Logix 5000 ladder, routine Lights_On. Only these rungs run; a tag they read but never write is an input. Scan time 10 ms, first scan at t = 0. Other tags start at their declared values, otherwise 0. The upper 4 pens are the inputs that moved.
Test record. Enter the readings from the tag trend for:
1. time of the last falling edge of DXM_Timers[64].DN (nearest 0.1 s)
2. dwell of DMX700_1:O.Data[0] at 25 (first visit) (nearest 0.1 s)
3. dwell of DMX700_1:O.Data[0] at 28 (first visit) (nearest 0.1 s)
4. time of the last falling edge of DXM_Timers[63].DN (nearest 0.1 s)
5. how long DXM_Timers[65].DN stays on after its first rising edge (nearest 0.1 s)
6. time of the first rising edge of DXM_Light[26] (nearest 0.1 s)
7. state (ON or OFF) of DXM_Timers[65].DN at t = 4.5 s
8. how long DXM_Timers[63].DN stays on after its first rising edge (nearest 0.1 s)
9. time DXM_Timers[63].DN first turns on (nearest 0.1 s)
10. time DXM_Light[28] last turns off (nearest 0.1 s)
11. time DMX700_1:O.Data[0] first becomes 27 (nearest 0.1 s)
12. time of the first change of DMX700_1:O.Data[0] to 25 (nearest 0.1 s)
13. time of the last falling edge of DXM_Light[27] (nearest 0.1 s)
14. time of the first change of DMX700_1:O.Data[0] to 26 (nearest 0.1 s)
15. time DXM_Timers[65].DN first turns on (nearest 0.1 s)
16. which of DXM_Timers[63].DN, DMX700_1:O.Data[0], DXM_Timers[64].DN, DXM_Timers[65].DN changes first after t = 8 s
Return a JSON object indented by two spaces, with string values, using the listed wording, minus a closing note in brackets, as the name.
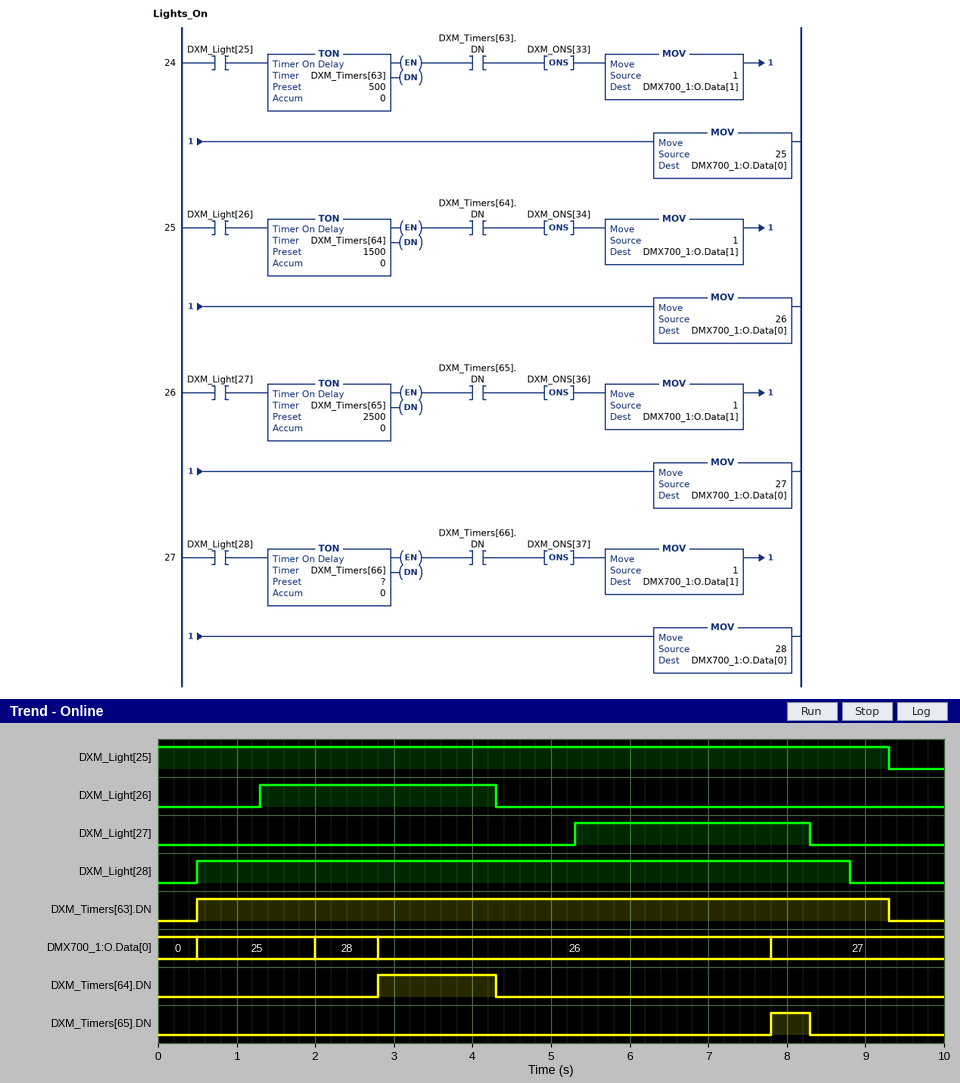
{
  "time of the last falling edge of DXM_Timers[64].DN": "4.3 s",
  "dwell of DMX700_1:O.Data[0] at 25 (first visit)": "1.5 s",
  "dwell of DMX700_1:O.Data[0] at 28 (first visit)": "0.8 s",
  "time of the last falling edge of DXM_Timers[63].DN": "9.3 s",
  "how long DXM_Timers[65].DN stays on after its first rising edge": "0.5 s",
  "time of the first rising edge of DXM_Light[26]": "1.3 s",
  "state (ON or OFF) of DXM_Timers[65].DN at t = 4.5 s": "OFF",
  "how long DXM_Timers[63].DN stays on after its first rising edge": "8.8 s",
  "time DXM_Timers[63].DN first turns on": "0.5 s",
  "time DXM_Light[28] last turns off": "8.8 s",
  "time DMX700_1:O.Data[0] first becomes 27": "7.8 s",
  "time of the first change of DMX700_1:O.Data[0] to 25": "0.5 s",
  "time of the last falling edge of DXM_Light[27]": "8.3 s",
  "time of the first change of DMX700_1:O.Data[0] to 26": "2.8 s",
  "time DXM_Timers[65].DN first turns on": "7.8 s",
  "which of DXM_Timers[63].DN, DMX700_1:O.Data[0], DXM_Timers[64].DN, DXM_Timers[65].DN changes first after t = 8 s": "DXM_Timers[65].DN"
}
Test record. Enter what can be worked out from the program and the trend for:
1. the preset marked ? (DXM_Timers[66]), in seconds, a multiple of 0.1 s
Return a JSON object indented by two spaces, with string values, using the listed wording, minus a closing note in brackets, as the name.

{
  "the preset marked ? (DXM_Timers[66]), in seconds, a multiple of 0.1 s": "1.5 s"
}
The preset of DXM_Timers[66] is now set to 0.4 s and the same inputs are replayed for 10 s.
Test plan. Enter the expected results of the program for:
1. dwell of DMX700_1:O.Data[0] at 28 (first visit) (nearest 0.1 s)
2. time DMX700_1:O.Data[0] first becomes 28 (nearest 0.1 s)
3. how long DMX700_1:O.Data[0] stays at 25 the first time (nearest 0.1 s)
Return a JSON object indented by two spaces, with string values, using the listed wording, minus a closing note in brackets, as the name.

{
  "dwell of DMX700_1:O.Data[0] at 28 (first visit)": "1.9 s",
  "time DMX700_1:O.Data[0] first becomes 28": "0.9 s",
  "how long DMX700_1:O.Data[0] stays at 25 the first time": "0.4 s"
}
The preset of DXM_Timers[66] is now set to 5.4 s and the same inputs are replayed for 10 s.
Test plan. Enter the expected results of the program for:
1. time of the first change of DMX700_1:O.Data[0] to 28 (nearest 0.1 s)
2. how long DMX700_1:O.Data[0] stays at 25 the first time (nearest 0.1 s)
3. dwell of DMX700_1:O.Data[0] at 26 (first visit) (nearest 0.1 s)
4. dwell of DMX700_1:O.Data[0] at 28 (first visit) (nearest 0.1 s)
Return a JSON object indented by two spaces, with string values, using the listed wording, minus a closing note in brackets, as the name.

{
  "time of the first change of DMX700_1:O.Data[0] to 28": "5.9 s",
  "how long DMX700_1:O.Data[0] stays at 25 the first time": "2.3 s",
  "dwell of DMX700_1:O.Data[0] at 26 (first visit)": "3.1 s",
  "dwell of DMX700_1:O.Data[0] at 28 (first visit)": "1.9 s"
}
